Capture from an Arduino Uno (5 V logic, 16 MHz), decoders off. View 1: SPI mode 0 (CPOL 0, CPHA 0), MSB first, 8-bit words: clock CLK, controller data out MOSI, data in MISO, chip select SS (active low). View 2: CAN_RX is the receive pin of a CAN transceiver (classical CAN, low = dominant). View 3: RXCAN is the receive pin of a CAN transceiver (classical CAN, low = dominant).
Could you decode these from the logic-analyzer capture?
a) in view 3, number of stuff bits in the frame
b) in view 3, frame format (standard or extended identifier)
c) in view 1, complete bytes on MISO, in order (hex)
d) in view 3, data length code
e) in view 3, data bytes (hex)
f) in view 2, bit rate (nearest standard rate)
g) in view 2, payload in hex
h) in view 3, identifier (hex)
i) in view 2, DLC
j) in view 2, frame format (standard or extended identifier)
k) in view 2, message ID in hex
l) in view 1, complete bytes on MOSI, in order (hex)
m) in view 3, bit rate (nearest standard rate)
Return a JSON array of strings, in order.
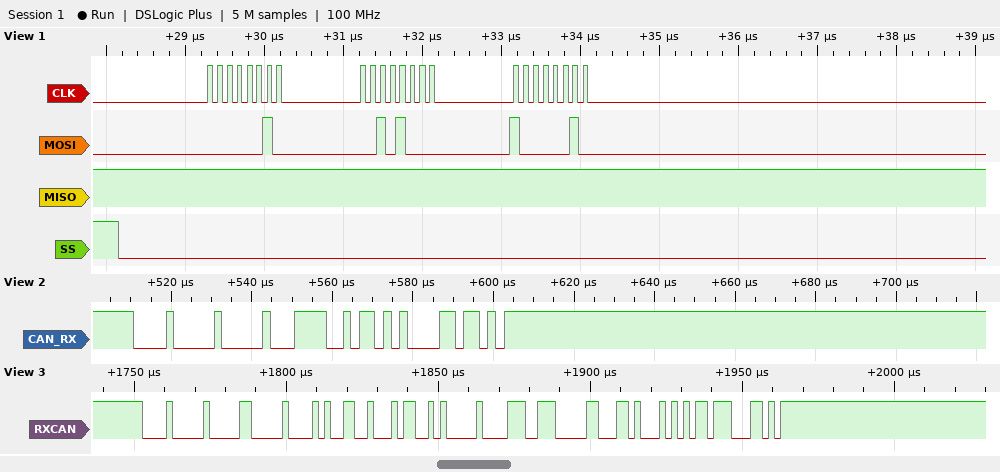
["5", "standard", "0xFF 0xFF 0xFF", "8", "02 99 16 50 07 38 23 45", "500 kbit/s", "E5", "0x080", "1", "standard", "0x080", "0x02 0x28 0x82", "500 kbit/s"]
